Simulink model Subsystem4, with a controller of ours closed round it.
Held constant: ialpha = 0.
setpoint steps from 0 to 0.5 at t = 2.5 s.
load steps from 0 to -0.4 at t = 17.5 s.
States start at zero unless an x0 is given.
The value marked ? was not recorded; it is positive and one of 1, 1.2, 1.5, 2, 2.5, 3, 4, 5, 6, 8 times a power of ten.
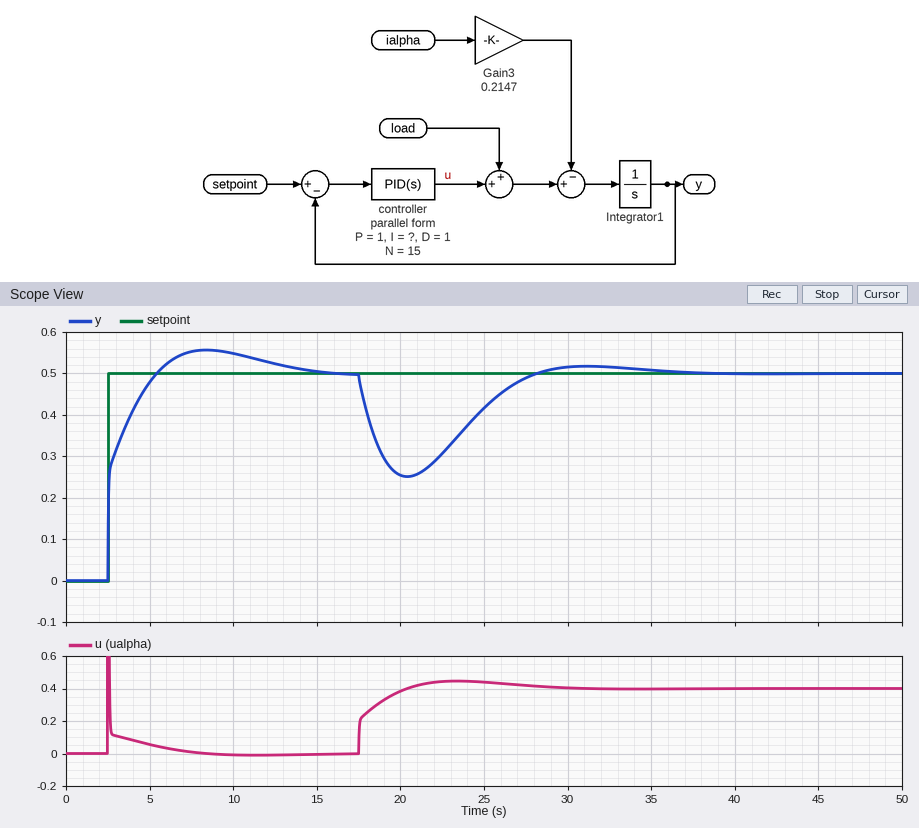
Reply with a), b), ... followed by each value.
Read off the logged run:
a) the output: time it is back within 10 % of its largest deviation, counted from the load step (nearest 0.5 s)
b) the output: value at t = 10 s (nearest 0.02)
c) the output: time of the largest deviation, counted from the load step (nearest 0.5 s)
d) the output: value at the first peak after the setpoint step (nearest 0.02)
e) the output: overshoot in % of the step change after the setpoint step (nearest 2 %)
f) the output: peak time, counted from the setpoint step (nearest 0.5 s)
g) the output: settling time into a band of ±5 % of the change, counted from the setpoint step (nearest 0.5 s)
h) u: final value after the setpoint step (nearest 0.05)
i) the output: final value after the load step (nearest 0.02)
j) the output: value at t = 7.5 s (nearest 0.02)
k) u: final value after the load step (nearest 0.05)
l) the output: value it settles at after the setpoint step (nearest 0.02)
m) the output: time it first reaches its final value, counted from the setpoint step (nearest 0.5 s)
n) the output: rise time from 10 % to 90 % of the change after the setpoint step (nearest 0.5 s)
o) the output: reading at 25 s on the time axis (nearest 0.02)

a) 9.5 s
b) 0.54
c) 3.0 s
d) 0.56
e) 12 %
f) 6.0 s
g) 10.0 s
h) 0.00
i) 0.50
j) 0.56
k) 0.40
l) 0.50
m) 3.0 s
n) 2.0 s
o) 0.42
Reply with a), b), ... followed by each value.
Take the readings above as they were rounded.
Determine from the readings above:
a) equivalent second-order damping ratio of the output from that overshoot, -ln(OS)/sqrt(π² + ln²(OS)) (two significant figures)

a) 0.56
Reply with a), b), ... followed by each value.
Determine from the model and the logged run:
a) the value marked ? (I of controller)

a) 0.3
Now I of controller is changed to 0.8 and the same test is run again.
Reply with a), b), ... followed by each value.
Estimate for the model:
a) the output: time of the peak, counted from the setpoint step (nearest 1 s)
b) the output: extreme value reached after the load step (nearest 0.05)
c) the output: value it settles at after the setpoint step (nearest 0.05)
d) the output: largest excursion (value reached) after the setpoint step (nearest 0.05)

a) 4 s
b) 0.30
c) 0.50
d) 0.60
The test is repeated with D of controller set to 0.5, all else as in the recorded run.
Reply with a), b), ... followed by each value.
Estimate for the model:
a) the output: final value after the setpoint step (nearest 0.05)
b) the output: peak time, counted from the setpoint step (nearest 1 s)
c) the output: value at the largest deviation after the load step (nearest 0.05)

a) 0.50
b) 5 s
c) 0.25
